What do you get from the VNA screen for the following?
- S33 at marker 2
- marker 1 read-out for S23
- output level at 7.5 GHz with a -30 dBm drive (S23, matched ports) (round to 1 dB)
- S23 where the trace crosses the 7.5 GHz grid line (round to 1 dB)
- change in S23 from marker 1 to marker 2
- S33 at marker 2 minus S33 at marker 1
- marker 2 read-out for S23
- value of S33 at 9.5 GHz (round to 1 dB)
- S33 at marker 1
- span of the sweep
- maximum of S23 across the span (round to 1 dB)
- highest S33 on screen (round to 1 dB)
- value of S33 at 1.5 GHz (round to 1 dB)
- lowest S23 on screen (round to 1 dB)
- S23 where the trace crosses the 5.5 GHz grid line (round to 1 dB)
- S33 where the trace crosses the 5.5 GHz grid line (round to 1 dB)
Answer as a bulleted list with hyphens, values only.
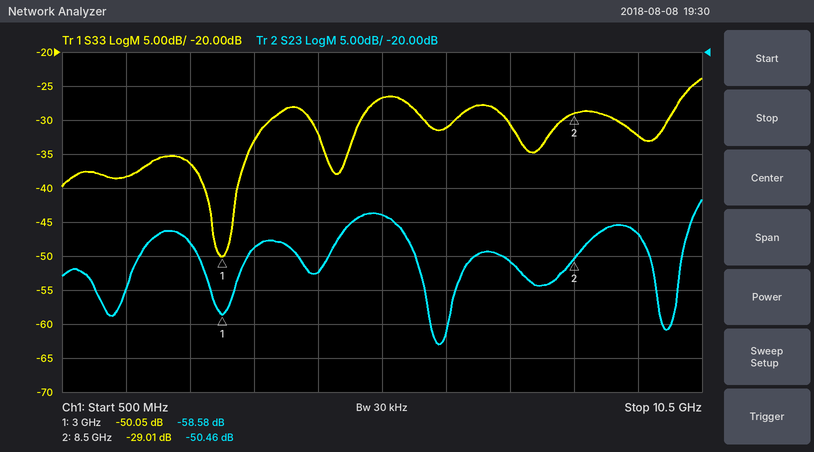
- -29.01 dB
- -58.58 dB
- -81 dBm
- -51 dB
- 8.12 dB
- 21.04 dB
- -50.46 dB
- -32 dB
- -50.05 dB
- 10 GHz
- -42 dB
- -24 dB
- -38 dB
- -63 dB
- -44 dB
- -27 dB
